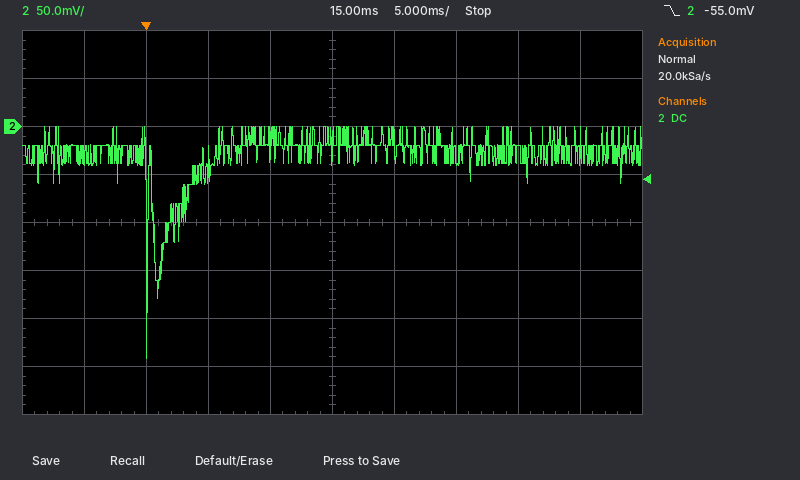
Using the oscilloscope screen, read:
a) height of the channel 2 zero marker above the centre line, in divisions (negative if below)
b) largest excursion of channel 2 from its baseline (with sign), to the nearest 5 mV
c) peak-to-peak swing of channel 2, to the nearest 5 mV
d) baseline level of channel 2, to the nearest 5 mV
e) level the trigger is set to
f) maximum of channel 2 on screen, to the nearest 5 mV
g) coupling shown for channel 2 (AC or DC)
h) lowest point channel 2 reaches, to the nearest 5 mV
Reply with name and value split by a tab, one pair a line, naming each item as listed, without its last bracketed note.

height of the channel 2 zero marker above the centre line, in divisions	+2.0 div
largest excursion of channel 2 from its baseline (with sign), to the nearest 5 mV	-215 mV
peak-to-peak swing of channel 2, to the nearest 5 mV	240 mV
baseline level of channel 2, to the nearest 5 mV	-25 mV
level the trigger is set to	-55.0 mV
maximum of channel 2 on screen, to the nearest 5 mV	0 mV
coupling shown for channel 2	DC
lowest point channel 2 reaches, to the nearest 5 mV	-240 mV
